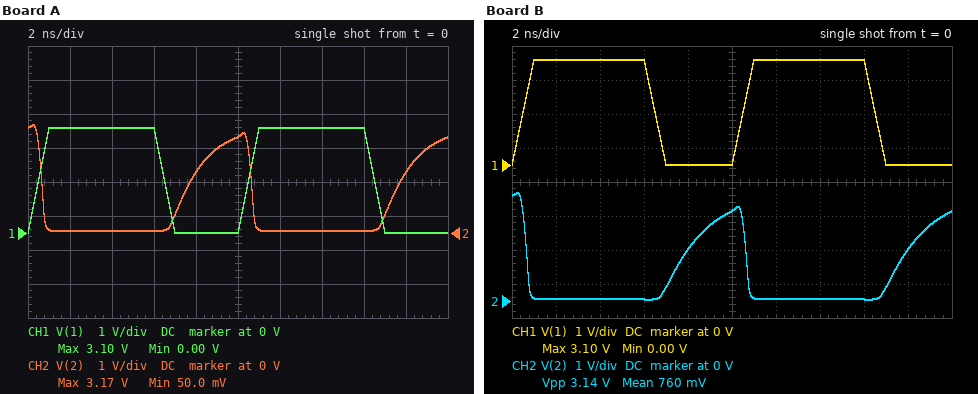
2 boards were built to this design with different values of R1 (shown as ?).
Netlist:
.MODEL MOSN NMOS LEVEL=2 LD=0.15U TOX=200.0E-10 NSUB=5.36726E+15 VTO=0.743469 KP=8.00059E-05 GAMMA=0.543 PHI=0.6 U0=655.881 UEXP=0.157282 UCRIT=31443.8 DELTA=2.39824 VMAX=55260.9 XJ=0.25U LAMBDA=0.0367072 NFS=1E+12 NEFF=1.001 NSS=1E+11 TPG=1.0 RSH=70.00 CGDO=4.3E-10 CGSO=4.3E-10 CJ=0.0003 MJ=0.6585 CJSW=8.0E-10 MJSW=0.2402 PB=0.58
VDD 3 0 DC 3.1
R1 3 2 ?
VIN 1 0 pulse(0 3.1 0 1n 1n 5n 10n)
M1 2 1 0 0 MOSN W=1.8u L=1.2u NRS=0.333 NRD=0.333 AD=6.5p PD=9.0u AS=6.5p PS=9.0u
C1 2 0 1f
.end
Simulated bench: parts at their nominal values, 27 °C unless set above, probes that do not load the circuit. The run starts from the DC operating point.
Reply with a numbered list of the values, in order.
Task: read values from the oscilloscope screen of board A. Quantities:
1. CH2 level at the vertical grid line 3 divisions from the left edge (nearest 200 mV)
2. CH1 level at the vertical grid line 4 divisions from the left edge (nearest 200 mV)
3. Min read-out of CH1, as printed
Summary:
1. 0 V
2. 0 V
3. 0.00 V
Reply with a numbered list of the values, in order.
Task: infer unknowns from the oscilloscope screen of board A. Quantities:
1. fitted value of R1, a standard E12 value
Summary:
1. 180 kΩ
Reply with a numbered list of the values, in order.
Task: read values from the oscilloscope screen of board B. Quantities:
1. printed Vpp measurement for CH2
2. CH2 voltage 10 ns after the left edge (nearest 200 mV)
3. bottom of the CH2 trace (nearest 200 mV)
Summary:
1. 3.14 V
2. 2.6 V
3. 0 V
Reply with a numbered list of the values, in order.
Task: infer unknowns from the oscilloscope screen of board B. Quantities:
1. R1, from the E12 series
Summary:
1. 220 kΩ
